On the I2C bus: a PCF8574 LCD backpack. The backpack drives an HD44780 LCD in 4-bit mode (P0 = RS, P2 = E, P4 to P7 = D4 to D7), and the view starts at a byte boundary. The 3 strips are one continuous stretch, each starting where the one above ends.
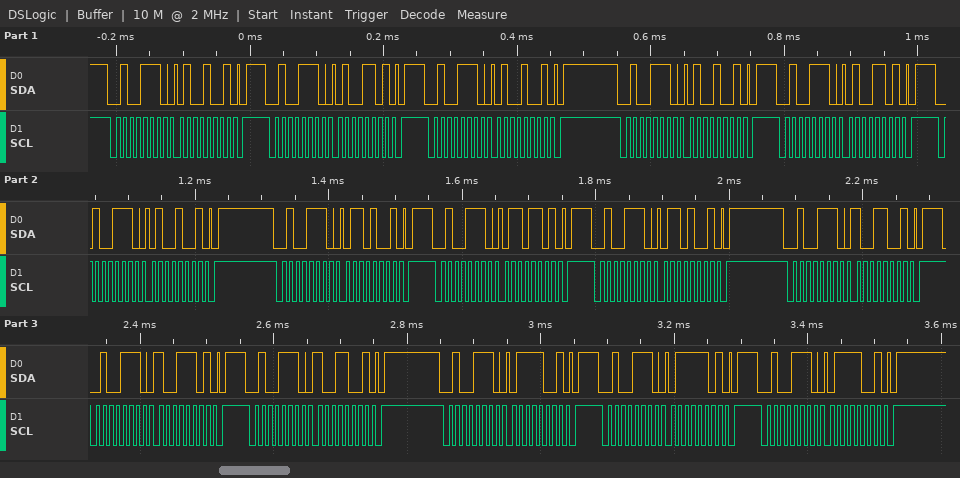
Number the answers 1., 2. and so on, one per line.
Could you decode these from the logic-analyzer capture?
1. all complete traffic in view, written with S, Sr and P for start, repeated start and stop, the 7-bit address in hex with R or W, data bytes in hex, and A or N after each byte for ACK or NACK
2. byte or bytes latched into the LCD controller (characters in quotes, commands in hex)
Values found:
1. S 27W A 49 A P S 27W A 4D A P S 27W A 49 A P S 27W A 49 A P S 27W A 4D A P S 27W A 49 A P S 27W A 69 A P S 27W A 6D A P S 27W A 69 A P S 27W A 99 A P S 27W A 9D A P S 27W A 99 A P S 27W A 79 A P S 27W A 7D A P S 27W A 79 A P
2. 'D' 'i'
